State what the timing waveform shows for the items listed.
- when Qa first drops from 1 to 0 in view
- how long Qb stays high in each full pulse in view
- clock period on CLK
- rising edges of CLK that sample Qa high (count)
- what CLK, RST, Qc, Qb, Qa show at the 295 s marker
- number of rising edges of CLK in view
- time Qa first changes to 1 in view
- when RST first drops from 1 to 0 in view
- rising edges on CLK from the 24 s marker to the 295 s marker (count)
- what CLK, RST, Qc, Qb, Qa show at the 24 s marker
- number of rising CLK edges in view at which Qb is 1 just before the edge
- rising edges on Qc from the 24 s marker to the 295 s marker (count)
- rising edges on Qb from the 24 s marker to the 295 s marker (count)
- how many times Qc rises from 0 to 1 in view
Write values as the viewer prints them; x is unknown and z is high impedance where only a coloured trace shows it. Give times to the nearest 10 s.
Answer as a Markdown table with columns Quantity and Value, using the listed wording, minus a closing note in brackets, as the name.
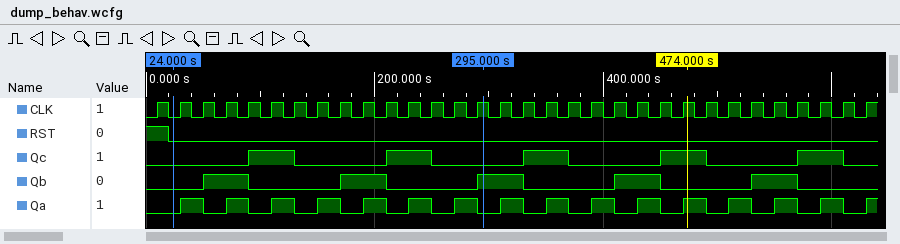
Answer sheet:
| Quantity | Value |
|---|---|
| when Qa first drops from 1 to 0 in view | 50 s |
| how long Qb stays high in each full pulse in view | 40 s, 40 s, 40 s, 40 s, 40 s |
| clock period on CLK | 20 s |
| rising edges of CLK that sample Qa high | 15 |
| what CLK, RST, Qc, Qb, Qa show at the 295 s marker | CLK=1, RST=0, Qc=0, Qb=1, Qa=0 |
| number of rising edges of CLK in view | 32 |
| time Qa first changes to 1 in view | 30 s |
| when RST first drops from 1 to 0 in view | 20 s |
| rising edges on CLK from the 24 s marker to the 295 s marker | 14 |
| what CLK, RST, Qc, Qb, Qa show at the 24 s marker | CLK=0, RST=0, Qc=0, Qb=0, Qa=0 |
| number of rising CLK edges in view at which Qb is 1 just before the edge | 10 |
| rising edges on Qc from the 24 s marker to the 295 s marker | 2 |
| rising edges on Qb from the 24 s marker to the 295 s marker | 3 |
| how many times Qc rises from 0 to 1 in view | 5 |
